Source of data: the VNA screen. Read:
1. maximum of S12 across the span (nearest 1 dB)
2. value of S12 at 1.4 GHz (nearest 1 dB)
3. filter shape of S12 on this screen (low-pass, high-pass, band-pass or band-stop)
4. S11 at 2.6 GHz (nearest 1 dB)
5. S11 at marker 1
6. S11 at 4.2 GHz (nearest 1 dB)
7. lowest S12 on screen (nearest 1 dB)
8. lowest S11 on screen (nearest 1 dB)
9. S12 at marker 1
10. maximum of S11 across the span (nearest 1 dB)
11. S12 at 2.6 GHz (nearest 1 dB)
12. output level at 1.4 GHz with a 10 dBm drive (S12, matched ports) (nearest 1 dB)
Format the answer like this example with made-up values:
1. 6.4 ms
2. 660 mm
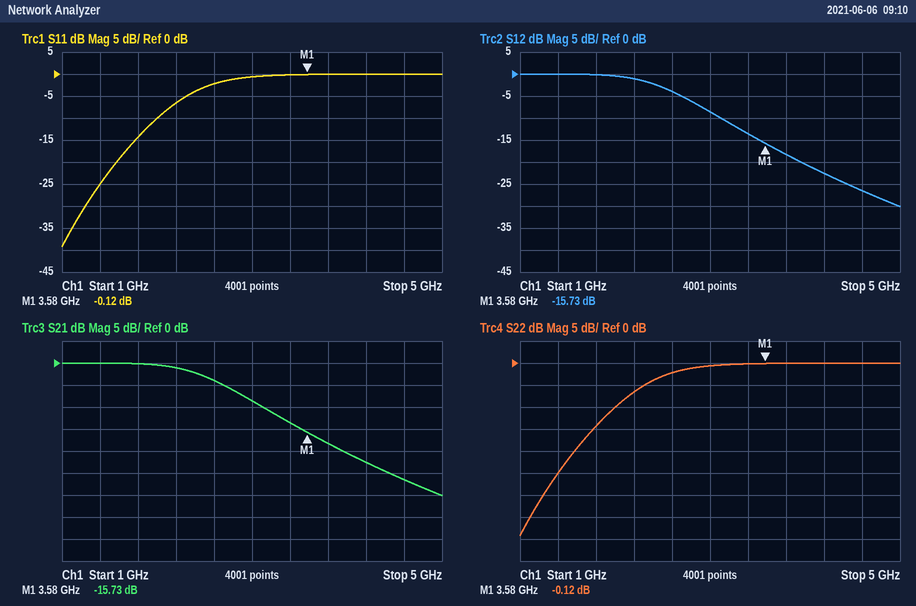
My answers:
1. 0 dB
2. 0 dB
3. low-pass
4. -2 dB
5. -0.12 dB
6. 0 dB
7. -30 dB
8. -39 dB
9. -15.73 dB
10. 0 dB
11. -4 dB
12. 10 dBm
